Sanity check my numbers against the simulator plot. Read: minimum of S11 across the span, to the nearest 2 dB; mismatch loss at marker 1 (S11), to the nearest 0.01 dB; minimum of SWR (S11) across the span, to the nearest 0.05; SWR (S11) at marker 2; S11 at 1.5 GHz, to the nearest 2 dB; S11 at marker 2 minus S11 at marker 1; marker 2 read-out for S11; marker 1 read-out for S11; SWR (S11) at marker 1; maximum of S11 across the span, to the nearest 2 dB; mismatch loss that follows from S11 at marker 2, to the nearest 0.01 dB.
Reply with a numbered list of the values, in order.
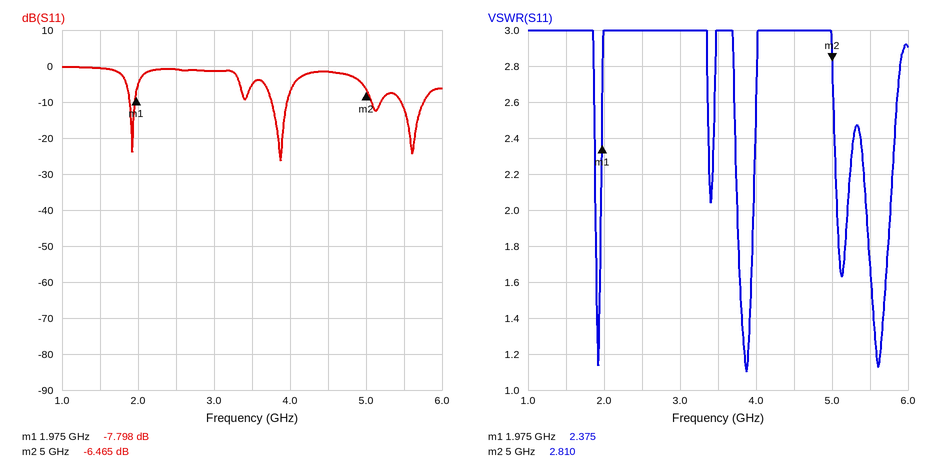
1. -26 dB
2. 0.79 dB
3. 1.10
4. 2.810
5. 0 dB
6. 1.333 dB
7. -6.465 dB
8. -7.798 dB
9. 2.375
10. 0 dB
11. 1.11 dB
